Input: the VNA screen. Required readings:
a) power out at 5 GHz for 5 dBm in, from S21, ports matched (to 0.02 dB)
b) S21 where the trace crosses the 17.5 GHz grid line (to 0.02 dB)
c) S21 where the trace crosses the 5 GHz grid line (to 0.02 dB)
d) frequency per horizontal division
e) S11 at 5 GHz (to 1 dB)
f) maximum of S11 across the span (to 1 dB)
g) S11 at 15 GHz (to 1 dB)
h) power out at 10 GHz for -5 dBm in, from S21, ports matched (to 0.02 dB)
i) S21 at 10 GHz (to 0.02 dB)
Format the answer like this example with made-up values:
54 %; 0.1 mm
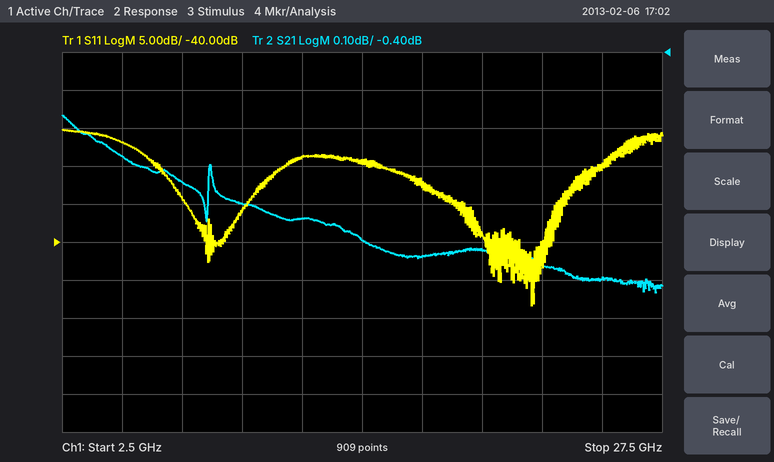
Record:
4.32 dBm; -0.94 dB; -0.68 dB; 2.5 GHz; -27 dB; -25 dB; -29 dB; -5.80 dBm; -0.80 dB
